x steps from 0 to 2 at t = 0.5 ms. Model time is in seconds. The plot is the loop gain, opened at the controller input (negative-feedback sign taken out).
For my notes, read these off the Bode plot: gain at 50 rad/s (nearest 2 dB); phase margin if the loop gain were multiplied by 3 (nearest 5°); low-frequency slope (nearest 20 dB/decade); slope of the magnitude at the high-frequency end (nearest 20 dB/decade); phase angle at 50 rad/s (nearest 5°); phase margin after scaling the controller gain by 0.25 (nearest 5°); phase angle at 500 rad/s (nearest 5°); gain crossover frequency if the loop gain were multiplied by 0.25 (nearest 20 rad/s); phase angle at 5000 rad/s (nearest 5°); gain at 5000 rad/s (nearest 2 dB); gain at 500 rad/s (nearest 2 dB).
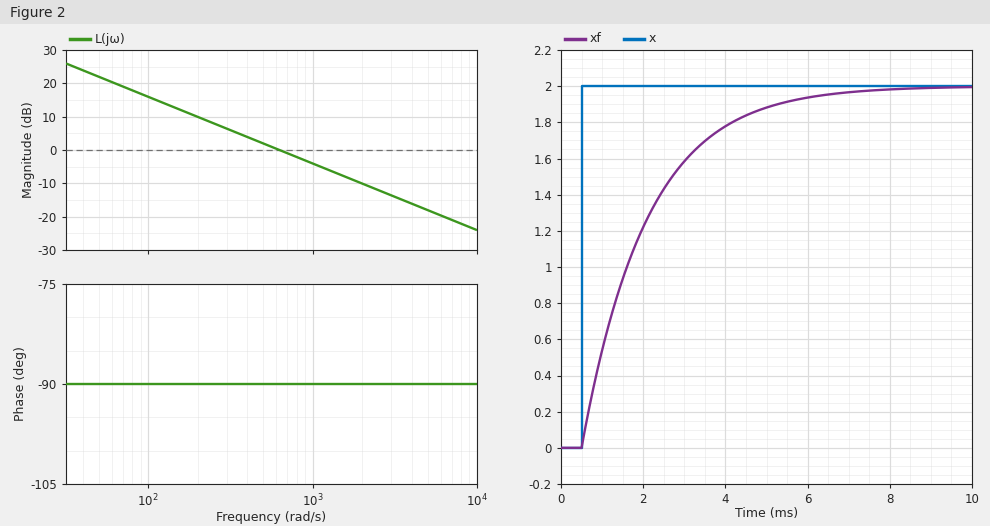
22 dB
90°
-20 dB/decade
-20 dB/decade
-90°
90°
-90°
160 rad/s
-90°
-18 dB
2 dB
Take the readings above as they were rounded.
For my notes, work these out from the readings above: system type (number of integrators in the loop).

1
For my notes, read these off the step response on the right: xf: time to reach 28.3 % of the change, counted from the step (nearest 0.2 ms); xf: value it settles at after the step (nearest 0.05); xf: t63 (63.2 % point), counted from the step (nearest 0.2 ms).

0.6 ms
2.00
1.6 ms
